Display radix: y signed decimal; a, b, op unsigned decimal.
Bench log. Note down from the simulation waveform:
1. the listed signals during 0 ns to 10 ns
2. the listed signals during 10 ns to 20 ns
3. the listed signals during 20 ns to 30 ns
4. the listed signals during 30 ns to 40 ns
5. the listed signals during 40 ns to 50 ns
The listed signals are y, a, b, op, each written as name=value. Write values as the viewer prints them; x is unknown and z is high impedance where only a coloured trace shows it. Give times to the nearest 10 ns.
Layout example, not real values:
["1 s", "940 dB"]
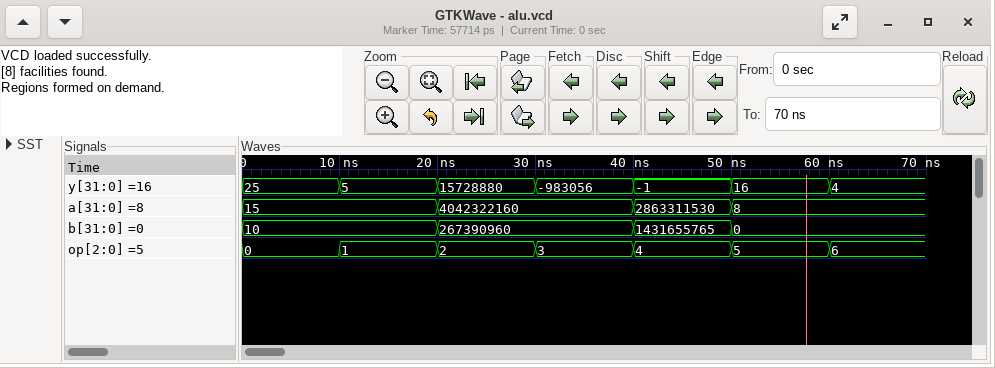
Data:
["y=25, a=15, b=10, op=0", "y=5, a=15, b=10, op=1", "y=15728880, a=4042322160, b=267390960, op=2", "y=-983056, a=4042322160, b=267390960, op=3", "y=-1, a=2863311530, b=1431655765, op=4"]
